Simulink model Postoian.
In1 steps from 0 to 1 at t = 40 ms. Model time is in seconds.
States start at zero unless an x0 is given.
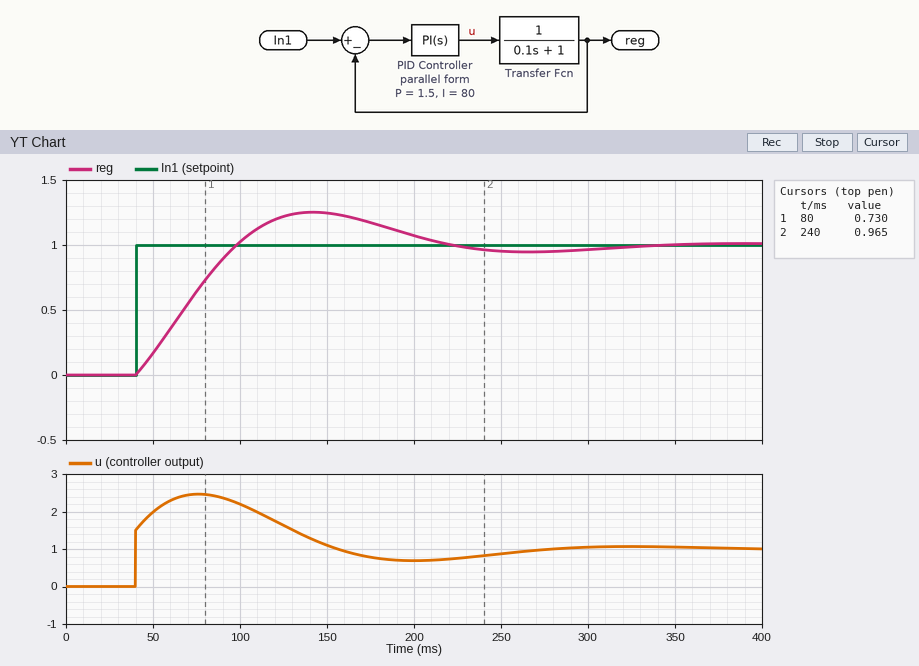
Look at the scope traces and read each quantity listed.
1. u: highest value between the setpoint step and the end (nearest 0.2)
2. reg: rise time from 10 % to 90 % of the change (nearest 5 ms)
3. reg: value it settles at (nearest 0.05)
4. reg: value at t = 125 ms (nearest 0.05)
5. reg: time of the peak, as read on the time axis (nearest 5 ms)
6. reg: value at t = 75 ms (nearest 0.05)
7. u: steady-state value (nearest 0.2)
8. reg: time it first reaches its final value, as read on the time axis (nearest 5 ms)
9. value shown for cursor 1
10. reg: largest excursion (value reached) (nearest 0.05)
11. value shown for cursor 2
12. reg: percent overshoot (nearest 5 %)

2.4
45 ms
1.00
1.20
140 ms
0.65
1.0
100 ms
0.730
1.25
0.965
25 %
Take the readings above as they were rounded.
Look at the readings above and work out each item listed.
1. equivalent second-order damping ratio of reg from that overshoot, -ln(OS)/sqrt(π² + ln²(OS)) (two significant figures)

0.40
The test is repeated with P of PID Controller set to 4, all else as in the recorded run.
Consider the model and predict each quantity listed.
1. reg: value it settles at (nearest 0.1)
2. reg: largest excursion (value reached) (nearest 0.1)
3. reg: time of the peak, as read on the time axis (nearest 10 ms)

1.0
1.1
130 ms
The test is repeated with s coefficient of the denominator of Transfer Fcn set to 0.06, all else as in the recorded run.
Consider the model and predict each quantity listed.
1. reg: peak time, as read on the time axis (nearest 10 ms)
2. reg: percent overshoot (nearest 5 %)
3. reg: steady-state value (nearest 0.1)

120 ms
15 %
1.0
